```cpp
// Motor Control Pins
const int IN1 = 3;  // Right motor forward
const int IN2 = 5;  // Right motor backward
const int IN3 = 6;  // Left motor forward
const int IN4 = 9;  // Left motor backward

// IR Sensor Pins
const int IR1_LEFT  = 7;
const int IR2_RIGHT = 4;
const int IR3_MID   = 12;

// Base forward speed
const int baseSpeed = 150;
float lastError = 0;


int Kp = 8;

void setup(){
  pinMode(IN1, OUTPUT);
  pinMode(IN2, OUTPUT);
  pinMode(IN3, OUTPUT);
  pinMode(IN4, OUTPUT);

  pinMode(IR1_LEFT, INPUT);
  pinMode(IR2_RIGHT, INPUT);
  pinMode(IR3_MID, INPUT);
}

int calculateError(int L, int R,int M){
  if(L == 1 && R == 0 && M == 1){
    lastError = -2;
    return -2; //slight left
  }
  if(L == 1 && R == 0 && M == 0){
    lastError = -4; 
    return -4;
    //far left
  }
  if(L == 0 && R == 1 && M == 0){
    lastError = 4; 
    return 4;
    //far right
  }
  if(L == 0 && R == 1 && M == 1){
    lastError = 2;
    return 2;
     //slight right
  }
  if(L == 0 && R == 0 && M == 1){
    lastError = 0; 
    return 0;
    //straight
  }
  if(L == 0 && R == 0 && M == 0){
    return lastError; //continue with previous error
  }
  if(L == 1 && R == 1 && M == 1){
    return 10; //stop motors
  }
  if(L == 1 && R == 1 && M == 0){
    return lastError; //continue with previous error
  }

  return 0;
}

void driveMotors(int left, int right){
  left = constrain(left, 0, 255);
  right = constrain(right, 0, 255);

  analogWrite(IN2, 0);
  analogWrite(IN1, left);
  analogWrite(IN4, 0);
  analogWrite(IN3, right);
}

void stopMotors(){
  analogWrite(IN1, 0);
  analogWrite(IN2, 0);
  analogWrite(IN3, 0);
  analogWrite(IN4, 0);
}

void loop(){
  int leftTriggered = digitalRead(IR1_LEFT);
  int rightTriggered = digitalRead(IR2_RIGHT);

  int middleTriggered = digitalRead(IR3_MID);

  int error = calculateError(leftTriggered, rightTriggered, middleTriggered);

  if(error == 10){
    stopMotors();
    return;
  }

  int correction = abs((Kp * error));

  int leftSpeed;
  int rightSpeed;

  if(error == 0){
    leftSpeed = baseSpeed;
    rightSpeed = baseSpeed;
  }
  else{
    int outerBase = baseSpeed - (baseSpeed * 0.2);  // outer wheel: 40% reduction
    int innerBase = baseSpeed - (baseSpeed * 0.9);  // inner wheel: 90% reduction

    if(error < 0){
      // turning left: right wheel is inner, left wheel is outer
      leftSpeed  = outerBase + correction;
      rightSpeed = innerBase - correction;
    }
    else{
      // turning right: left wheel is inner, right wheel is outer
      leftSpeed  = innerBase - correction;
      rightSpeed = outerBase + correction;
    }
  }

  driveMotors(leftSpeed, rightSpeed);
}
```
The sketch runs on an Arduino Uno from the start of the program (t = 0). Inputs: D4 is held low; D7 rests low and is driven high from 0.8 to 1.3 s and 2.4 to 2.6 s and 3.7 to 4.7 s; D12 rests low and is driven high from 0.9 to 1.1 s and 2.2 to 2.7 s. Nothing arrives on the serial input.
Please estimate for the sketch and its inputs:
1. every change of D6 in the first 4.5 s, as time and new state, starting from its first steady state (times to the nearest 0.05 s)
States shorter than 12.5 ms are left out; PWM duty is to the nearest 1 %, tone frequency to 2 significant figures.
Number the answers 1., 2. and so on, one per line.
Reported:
1. 0 s PWM 59 %; 0.8 s low; 2.2 s PWM 59 %; 2.4 s low; 2.6 s PWM 59 %; 3.7 s low
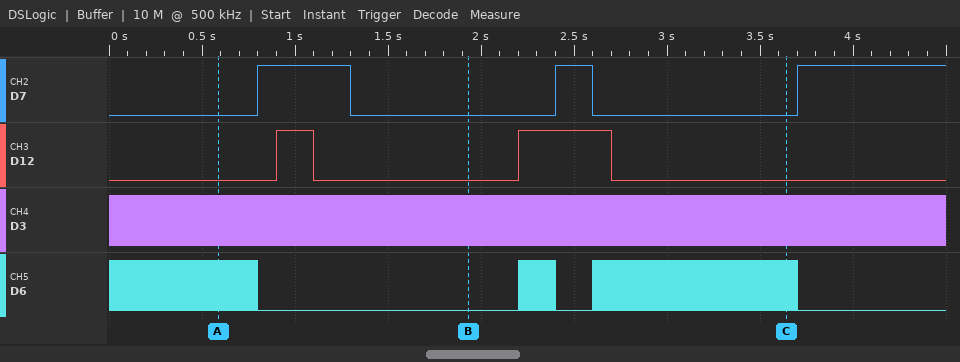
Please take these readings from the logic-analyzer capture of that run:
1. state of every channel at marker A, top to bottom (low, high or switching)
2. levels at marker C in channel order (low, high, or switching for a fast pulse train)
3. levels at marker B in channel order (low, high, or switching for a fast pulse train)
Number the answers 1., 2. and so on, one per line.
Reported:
1. D7 low, D12 low, D3 switching, D6 switching
2. D7 low, D12 low, D3 switching, D6 switching
3. D7 low, D12 low, D3 switching, D6 low
